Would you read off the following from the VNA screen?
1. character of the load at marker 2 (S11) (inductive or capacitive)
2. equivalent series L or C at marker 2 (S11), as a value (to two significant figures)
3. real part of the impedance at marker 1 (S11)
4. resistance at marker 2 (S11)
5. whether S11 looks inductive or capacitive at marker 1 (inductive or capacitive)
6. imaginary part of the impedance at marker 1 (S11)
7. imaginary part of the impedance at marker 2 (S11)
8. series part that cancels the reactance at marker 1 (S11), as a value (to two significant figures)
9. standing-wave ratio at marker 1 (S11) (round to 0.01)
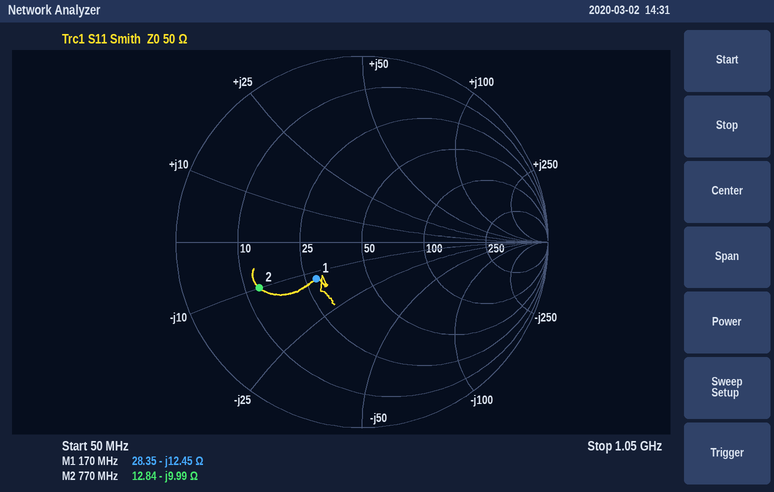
capacitive
21 pF
28.35 Ω
12.84 Ω
capacitive
-12.45 Ω
-9.99 Ω
12 nH
1.92
